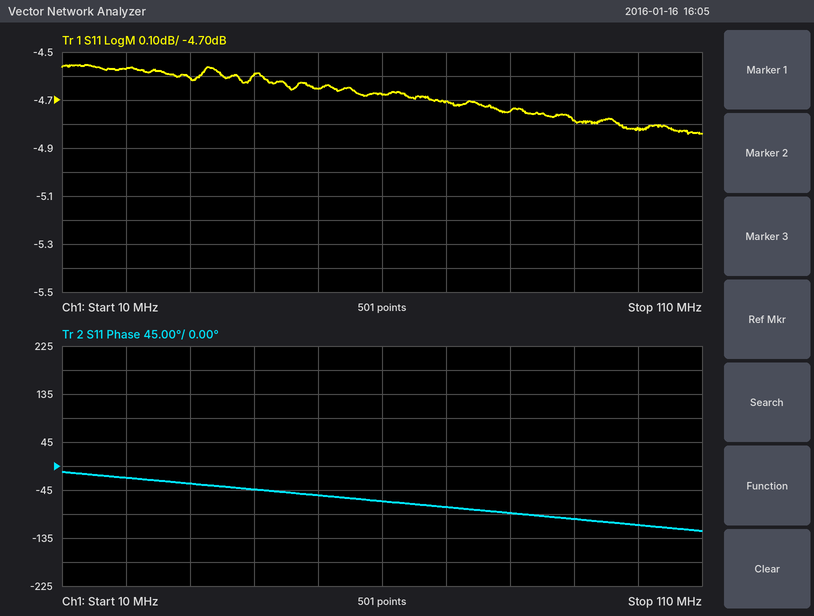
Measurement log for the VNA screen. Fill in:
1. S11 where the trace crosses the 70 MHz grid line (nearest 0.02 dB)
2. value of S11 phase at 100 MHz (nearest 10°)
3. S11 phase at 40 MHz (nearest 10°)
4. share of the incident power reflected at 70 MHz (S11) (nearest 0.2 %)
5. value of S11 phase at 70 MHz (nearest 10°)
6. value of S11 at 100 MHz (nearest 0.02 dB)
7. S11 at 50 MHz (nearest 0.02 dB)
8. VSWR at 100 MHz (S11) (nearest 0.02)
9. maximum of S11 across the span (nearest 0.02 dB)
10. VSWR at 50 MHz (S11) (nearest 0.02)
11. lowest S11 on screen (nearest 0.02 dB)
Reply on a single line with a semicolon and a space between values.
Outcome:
-4.70 dB; -110°; -40°; 33.8 %; -80°; -4.82 dB; -4.66 dB; 3.70; -4.56 dB; 3.82; -4.84 dB
